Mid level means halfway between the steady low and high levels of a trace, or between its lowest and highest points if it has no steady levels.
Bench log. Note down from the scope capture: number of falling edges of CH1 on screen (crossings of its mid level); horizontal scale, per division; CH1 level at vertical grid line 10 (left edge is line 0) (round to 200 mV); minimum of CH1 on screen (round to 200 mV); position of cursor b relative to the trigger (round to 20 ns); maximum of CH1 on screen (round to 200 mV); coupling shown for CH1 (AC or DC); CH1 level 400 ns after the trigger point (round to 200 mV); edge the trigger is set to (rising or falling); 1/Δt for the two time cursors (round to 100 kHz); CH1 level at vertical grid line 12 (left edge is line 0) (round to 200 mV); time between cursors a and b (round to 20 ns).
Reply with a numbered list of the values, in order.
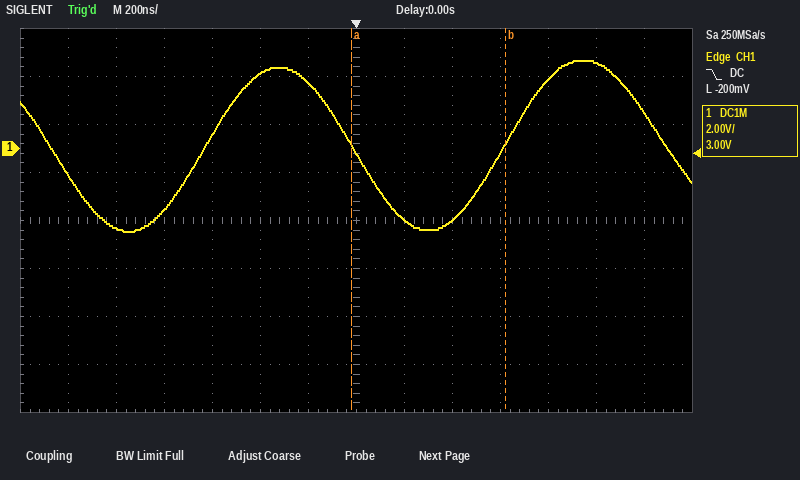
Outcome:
1. 3
2. 200 ns
3. -200 mV
4. -3.4 V
5. +620 ns
6. 3.6 V
7. DC
8. -3.0 V
9. falling
10. 1.6 MHz
11. 3.6 V
12. 640 ns
